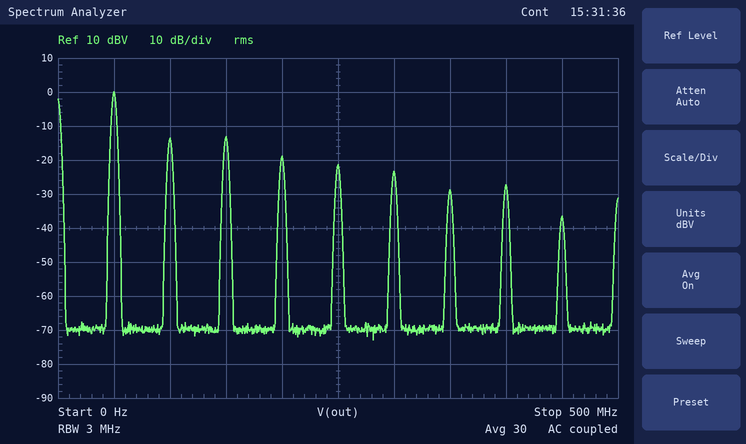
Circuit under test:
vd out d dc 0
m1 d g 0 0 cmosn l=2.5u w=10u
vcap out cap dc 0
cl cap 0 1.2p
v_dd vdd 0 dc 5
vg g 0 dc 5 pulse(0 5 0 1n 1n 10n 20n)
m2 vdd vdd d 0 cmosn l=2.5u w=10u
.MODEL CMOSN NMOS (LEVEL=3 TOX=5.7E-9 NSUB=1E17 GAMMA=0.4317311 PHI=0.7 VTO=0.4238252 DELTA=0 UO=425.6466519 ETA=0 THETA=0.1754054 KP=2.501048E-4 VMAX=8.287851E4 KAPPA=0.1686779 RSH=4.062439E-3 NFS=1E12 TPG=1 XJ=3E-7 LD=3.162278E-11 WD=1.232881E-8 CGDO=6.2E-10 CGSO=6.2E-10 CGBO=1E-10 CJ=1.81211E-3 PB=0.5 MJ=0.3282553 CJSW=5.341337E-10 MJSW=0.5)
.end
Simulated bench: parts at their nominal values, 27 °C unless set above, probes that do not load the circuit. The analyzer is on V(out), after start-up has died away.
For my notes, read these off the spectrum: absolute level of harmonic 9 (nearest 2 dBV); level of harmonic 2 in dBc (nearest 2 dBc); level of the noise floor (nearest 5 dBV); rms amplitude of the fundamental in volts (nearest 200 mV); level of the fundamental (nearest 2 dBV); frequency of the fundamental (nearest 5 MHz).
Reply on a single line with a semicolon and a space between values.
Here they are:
-36 dBV; -14 dBc; -70 dBV; 1.0 V; 0 dBV; 50 MHz
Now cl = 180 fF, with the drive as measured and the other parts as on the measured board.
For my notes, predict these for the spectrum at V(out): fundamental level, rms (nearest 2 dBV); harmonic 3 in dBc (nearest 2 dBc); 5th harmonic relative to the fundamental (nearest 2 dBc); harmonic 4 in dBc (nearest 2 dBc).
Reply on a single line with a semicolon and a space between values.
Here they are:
2 dBV; -12 dBc; -20 dBc; -16 dBc
